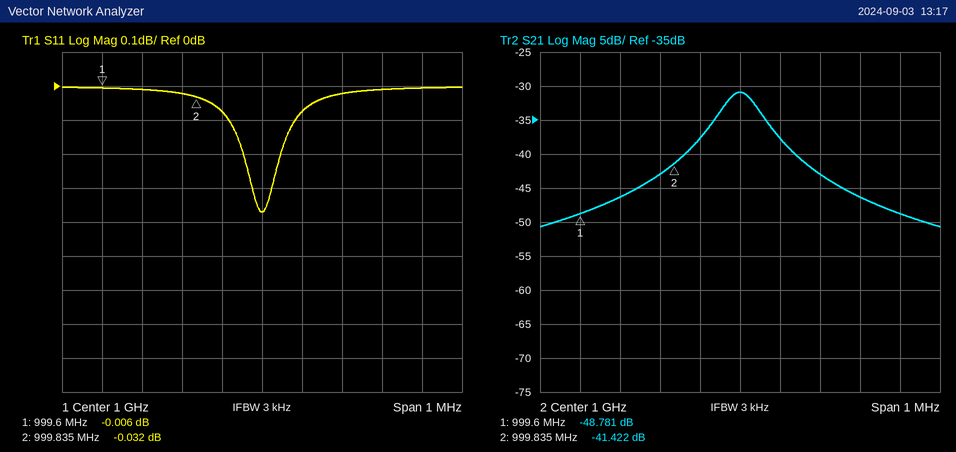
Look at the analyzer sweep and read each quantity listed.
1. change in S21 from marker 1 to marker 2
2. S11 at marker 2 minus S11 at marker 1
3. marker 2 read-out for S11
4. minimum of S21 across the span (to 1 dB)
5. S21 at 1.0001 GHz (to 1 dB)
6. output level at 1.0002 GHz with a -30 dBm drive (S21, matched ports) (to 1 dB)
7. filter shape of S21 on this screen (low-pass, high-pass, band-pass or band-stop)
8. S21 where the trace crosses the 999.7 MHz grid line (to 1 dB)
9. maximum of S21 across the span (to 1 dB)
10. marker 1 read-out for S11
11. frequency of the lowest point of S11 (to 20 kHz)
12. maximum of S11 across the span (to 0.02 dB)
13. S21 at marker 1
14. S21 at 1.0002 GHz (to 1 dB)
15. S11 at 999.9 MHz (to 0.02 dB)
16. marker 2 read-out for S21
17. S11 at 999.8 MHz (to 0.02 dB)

7.359 dB
-0.026 dB
-0.032 dB
-51 dB
-38 dB
-73 dBm
band-pass
-46 dB
-31 dB
-0.006 dB
1.00000 GHz
0.00 dB
-48.781 dB
-43 dB
-0.08 dB
-41.422 dB
-0.02 dB
